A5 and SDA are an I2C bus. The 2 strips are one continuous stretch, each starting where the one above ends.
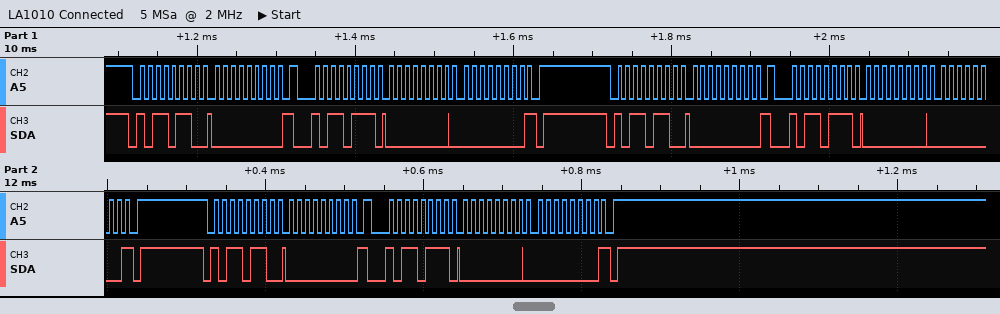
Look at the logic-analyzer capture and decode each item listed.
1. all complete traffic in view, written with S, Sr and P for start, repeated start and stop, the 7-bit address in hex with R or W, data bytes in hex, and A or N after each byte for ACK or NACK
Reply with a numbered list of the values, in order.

1. S 5BW A 00 A Sr 5BR A 00 A 00 N P S 5BW A 00 A Sr 5BR A 00 A 00 N P S 5BW A 00 A Sr 5BR A 00 A 00 N P
